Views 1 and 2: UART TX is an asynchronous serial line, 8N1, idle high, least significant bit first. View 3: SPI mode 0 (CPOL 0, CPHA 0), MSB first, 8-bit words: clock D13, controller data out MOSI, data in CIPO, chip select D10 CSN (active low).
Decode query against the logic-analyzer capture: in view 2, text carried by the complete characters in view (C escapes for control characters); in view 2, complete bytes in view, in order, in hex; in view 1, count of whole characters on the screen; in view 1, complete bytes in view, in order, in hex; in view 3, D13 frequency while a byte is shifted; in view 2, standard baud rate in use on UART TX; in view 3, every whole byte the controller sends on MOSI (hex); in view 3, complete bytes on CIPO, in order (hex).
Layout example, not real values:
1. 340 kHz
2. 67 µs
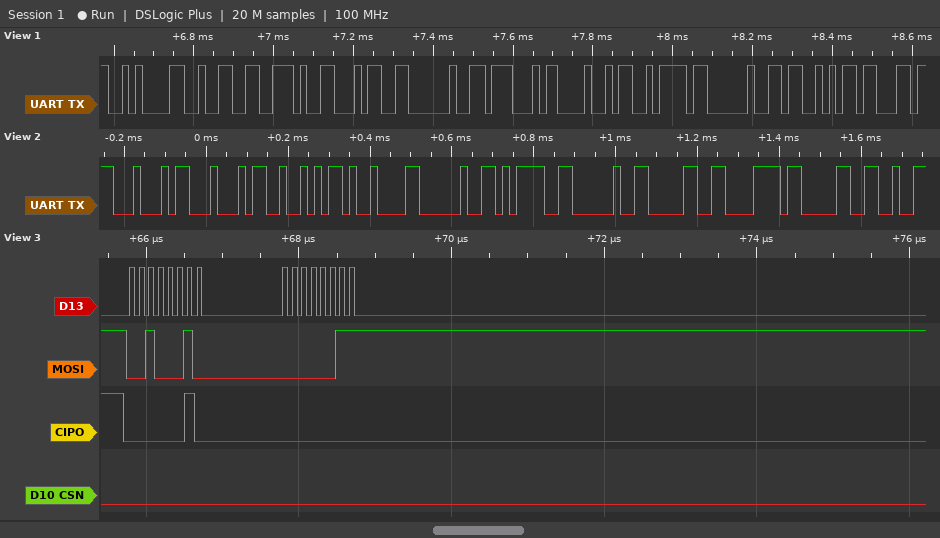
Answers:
1. "DDR\t = 0x0"
2. 0x44 0x44 0x52 0x09 0x20 0x3D 0x20 0x30 0x78 0x30
3. 11
4. 0A 32 2E 34 20 47 48 7A 20 53 63
5. 8 MHz
6. 57600 baud
7. 22 03
8. 02 00
